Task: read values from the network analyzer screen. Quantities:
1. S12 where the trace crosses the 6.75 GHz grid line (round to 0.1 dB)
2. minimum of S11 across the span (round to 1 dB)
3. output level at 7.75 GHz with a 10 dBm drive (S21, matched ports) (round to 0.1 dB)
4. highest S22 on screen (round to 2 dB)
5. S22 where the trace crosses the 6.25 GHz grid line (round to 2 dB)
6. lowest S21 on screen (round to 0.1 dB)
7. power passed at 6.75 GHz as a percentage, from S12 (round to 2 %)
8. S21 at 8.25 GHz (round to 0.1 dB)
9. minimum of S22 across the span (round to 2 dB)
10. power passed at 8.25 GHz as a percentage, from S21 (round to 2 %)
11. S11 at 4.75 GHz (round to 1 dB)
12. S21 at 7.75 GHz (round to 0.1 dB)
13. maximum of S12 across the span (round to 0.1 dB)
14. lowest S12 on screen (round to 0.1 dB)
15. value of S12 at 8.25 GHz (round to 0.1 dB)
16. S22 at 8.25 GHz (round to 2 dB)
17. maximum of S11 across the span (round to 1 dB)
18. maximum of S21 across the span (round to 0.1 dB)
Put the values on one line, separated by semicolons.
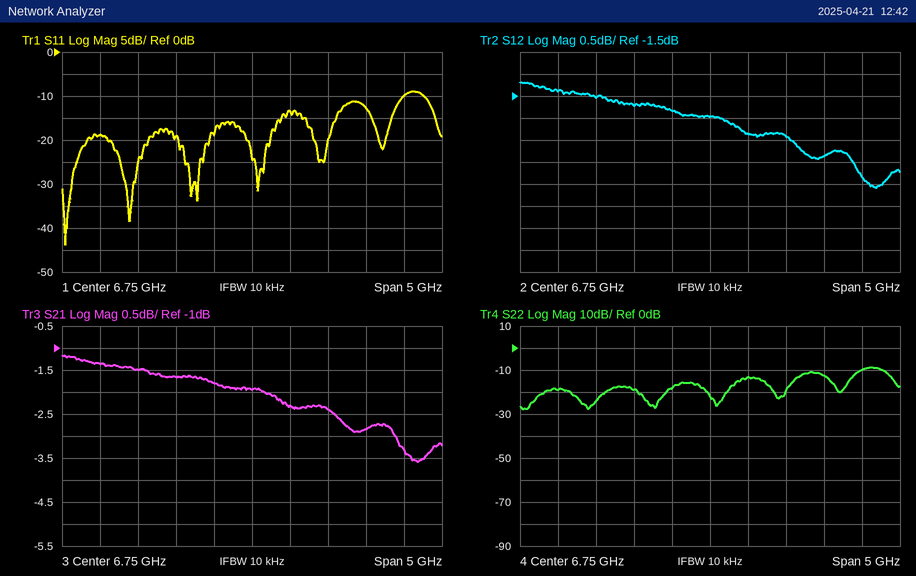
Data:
-2.0 dB; -44 dB; 7.6 dBm; -8 dB; -18 dB; -3.6 dB; 64 %; -2.8 dB; -28 dB; 52 %; -19 dB; -2.4 dB; -1.2 dB; -3.6 dB; -2.9 dB; -12 dB; -9 dB; -1.2 dB
